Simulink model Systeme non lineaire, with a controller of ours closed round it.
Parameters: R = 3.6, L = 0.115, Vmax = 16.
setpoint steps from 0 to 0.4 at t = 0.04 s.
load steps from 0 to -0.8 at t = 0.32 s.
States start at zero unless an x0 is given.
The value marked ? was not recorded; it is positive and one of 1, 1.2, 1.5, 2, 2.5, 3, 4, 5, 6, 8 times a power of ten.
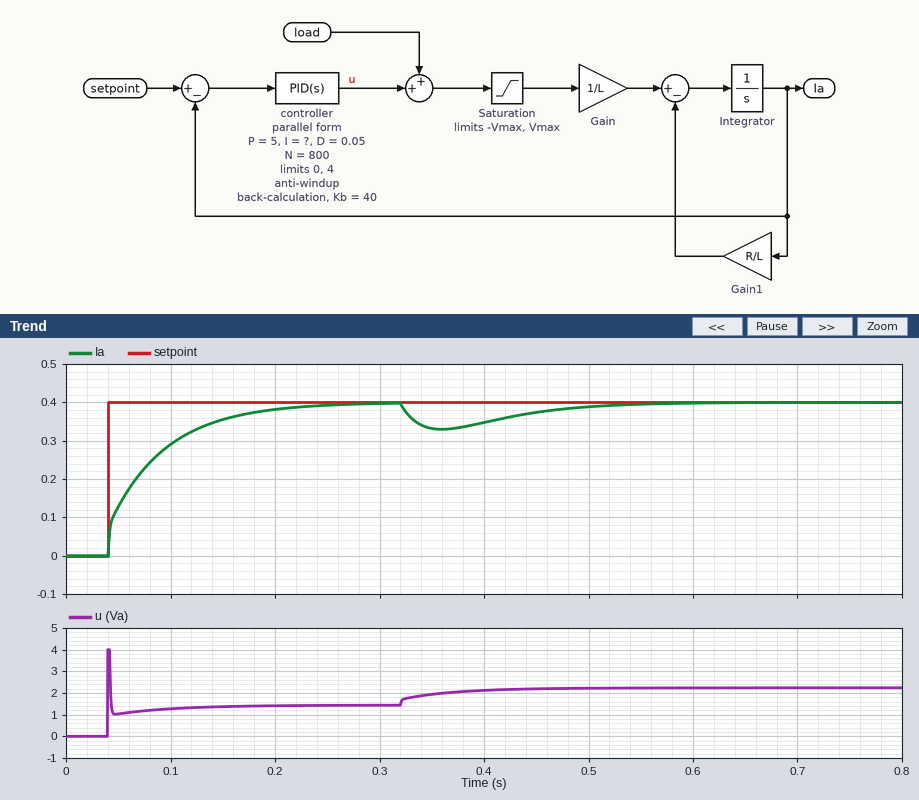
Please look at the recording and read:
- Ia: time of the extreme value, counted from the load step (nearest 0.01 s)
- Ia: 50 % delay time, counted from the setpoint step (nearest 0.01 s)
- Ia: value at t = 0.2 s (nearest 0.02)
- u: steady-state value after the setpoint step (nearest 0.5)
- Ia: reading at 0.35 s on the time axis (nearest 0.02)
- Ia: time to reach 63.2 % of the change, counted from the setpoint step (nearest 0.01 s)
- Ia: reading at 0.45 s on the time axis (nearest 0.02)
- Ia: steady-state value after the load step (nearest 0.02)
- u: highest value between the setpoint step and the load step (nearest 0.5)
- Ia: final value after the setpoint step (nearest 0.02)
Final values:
0.04 s
0.03 s
0.38
1.5
0.34
0.04 s
0.38
0.40
4.0
0.40
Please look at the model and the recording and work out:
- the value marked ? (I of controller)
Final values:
100
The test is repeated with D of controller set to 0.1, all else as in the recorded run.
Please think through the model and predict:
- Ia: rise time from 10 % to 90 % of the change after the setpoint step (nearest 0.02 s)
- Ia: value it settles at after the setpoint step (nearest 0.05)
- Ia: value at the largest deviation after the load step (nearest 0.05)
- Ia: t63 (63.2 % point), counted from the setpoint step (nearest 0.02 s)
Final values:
0.14 s
0.40
0.35
0.06 s
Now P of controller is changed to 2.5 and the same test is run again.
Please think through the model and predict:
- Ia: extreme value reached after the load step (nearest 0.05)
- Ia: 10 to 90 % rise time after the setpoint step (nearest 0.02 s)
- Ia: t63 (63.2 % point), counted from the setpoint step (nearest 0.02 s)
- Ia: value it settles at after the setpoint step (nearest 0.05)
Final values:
0.30
0.10 s
0.06 s
0.40
